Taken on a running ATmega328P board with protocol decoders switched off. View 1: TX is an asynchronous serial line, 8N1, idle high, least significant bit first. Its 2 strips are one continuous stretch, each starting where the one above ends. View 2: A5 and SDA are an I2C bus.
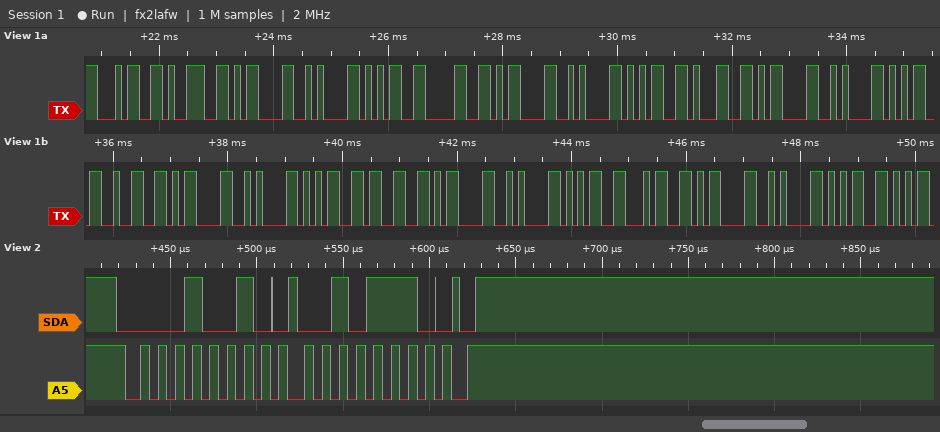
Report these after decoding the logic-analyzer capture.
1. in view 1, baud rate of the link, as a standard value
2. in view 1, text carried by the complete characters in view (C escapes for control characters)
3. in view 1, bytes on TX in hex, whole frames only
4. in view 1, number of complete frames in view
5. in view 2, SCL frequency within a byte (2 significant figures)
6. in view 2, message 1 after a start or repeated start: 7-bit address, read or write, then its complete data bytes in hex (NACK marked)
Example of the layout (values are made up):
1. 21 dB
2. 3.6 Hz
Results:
1. 9600 baud
2. "49\r\n50\r\n51\r\n52\r\n53\r\n54\r\n5"
3. 34 39 0D 0A 35 30 0D 0A 35 31 0D 0A 35 32 0D 0A 35 33 0D 0A 35 34 0D 0A 35
4. 25
5. 100 kHz
6. 0x09 write: 2E
